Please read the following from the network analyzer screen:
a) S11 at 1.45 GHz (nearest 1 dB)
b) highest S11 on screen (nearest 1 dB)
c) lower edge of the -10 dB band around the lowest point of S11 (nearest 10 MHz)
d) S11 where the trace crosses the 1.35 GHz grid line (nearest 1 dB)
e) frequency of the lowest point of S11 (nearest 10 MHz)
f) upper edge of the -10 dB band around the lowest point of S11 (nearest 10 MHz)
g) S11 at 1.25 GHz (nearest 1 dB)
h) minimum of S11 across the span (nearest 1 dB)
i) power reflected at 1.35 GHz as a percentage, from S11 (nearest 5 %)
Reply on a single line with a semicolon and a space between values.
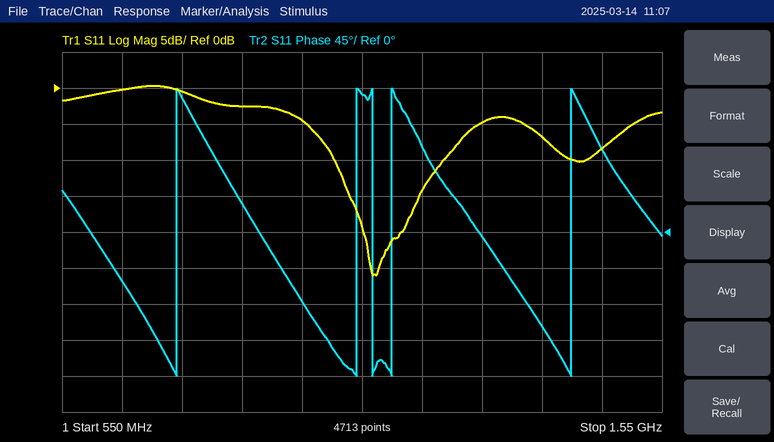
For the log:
-8 dB; 0 dB; 1.00 GHz; -7 dB; 1.07 GHz; 1.19 GHz; -5 dB; -26 dB; 20 %
